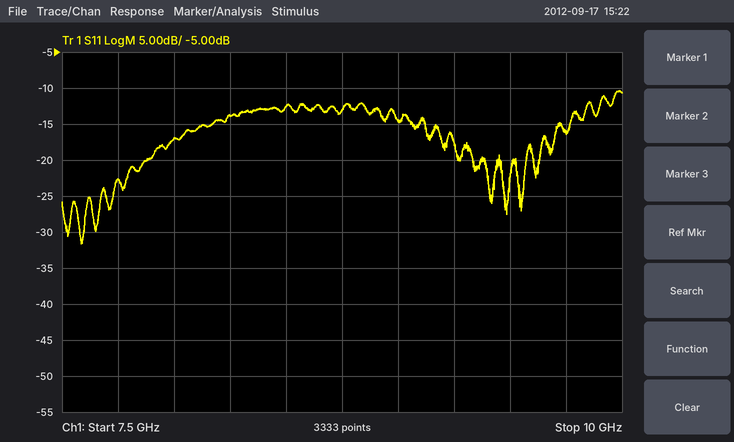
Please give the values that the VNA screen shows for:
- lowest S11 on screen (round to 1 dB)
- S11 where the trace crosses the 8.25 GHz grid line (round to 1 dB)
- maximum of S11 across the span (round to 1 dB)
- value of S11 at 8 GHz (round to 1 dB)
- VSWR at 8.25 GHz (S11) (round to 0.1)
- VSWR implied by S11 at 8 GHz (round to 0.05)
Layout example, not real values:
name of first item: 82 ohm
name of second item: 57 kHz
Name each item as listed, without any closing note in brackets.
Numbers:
lowest S11 on screen: -32 dB
S11 where the trace crosses the 8.25 GHz grid line: -14 dB
maximum of S11 across the span: -10 dB
value of S11 at 8 GHz: -17 dB
VSWR at 8.25 GHz (S11): 1.5
VSWR implied by S11 at 8 GHz: 1.35
